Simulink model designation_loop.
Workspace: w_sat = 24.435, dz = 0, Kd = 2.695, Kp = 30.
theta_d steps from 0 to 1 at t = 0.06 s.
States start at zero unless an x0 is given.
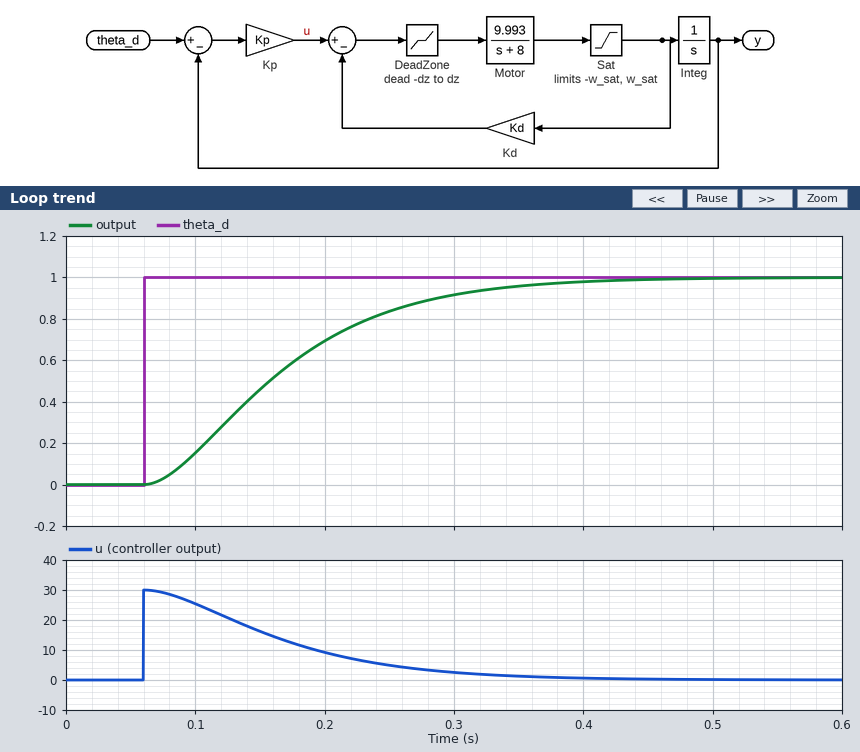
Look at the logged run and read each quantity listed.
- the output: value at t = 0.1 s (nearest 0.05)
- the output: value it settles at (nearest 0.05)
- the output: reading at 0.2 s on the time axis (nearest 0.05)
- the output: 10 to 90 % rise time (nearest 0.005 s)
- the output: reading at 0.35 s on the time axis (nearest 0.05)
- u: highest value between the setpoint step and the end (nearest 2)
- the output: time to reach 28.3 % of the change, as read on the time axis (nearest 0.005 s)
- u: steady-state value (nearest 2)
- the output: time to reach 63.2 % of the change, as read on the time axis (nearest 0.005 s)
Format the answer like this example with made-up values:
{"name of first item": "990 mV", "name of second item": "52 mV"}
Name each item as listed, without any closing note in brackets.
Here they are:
{"the output: value at t = 0.1 s": "0.15", "the output: value it settles at": "1.00", "the output: reading at 0.2 s on the time axis": "0.70", "the output: 10 to 90 % rise time": "0.195 s", "the output: reading at 0.35 s on the time axis": "0.95", "u: highest value between the setpoint step and the end": "30", "the output: time to reach 28.3 % of the change, as read on the time axis": "0.120 s", "u: steady-state value": "0", "the output: time to reach 63.2 % of the change, as read on the time axis": "0.185 s"}
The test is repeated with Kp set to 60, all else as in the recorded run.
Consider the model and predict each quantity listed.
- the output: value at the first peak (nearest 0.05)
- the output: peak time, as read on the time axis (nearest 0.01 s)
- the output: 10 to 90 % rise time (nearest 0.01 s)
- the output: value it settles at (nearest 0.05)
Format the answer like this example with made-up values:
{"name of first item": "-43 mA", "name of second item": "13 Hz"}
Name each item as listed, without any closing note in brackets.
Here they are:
{"the output: value at the first peak": "1.05", "the output: peak time, as read on the time axis": "0.24 s", "the output: 10 to 90 % rise time": "0.09 s", "the output: value it settles at": "1.00"}
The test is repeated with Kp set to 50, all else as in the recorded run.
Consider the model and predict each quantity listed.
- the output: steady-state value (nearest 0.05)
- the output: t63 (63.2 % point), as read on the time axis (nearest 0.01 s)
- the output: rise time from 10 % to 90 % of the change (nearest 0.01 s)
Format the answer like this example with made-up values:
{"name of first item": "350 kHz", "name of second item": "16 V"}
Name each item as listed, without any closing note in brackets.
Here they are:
{"the output: steady-state value": "1.00", "the output: t63 (63.2 % point), as read on the time axis": "0.14 s", "the output: rise time from 10 % to 90 % of the change": "0.11 s"}
